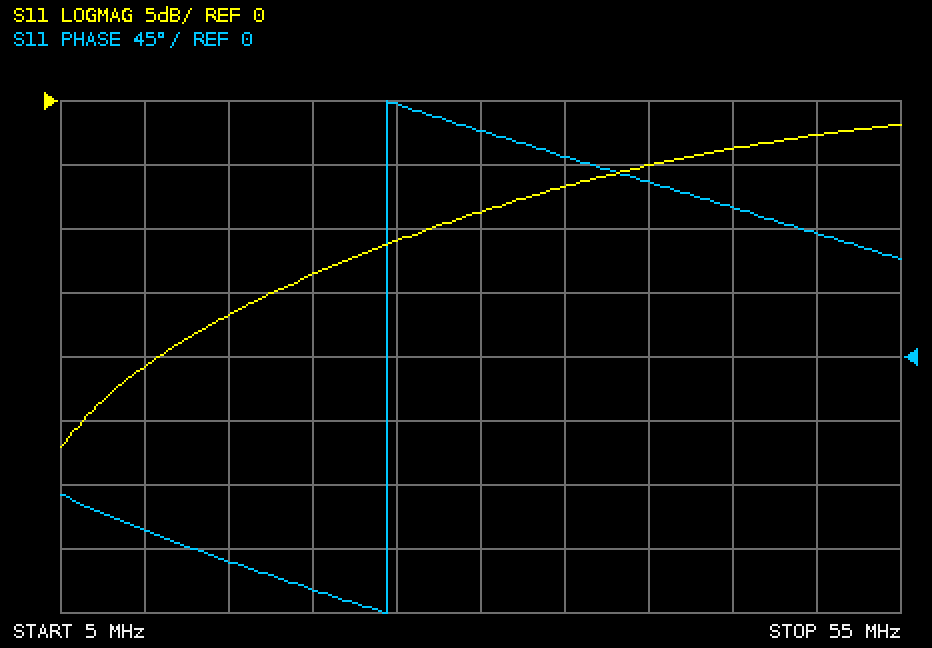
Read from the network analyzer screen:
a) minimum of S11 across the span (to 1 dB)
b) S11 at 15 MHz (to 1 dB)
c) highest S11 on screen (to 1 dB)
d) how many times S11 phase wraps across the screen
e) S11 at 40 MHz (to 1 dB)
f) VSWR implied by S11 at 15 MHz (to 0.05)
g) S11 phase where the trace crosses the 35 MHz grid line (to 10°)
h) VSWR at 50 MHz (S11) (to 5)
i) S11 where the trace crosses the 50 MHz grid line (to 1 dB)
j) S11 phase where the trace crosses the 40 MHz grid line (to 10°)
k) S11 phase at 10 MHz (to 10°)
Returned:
-27 dB
-17 dB
-2 dB
1
-5 dB
1.35
140°
5
-3 dB
120°
-120°
